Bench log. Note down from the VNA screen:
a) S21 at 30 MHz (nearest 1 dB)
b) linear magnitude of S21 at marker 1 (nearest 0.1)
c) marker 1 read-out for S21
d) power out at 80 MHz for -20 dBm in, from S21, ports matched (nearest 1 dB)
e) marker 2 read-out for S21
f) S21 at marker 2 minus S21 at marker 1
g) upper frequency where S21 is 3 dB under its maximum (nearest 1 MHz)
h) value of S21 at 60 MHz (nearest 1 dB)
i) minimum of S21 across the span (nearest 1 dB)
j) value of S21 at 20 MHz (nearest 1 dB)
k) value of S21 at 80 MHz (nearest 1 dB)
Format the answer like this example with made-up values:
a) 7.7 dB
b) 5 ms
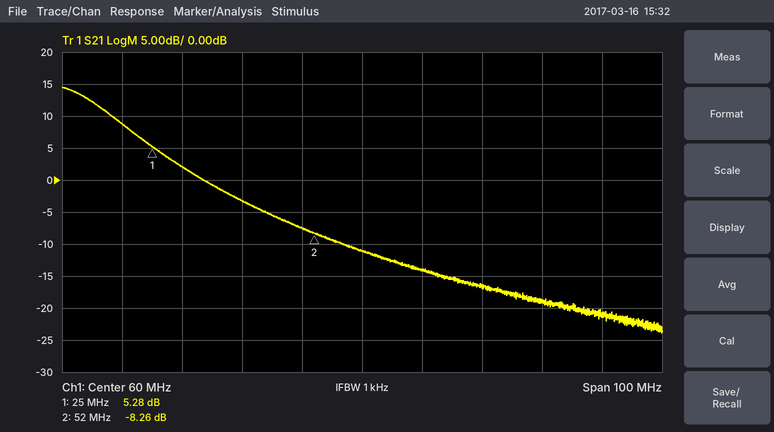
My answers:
a) 2 dB
b) 1.8
c) 5.28 dB
d) -37 dBm
e) -8.26 dB
f) -13.54 dB
g) 16 MHz
h) -11 dB
i) -24 dB
j) 9 dB
k) -17 dB
